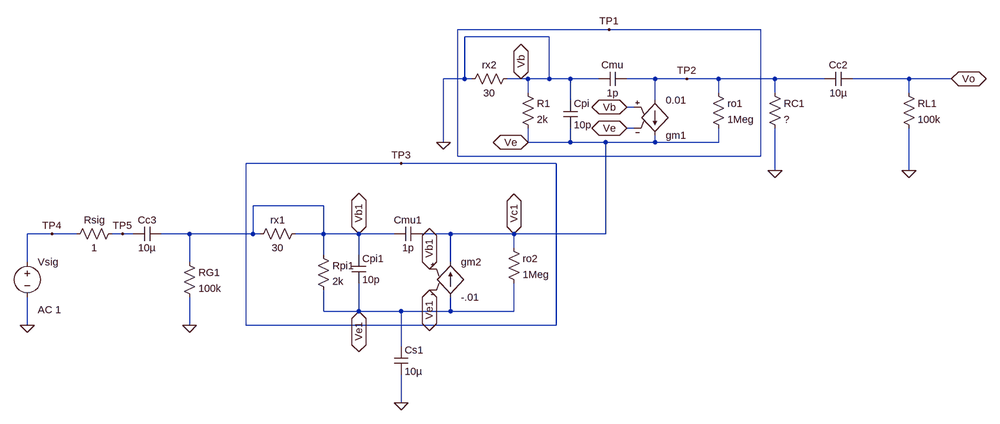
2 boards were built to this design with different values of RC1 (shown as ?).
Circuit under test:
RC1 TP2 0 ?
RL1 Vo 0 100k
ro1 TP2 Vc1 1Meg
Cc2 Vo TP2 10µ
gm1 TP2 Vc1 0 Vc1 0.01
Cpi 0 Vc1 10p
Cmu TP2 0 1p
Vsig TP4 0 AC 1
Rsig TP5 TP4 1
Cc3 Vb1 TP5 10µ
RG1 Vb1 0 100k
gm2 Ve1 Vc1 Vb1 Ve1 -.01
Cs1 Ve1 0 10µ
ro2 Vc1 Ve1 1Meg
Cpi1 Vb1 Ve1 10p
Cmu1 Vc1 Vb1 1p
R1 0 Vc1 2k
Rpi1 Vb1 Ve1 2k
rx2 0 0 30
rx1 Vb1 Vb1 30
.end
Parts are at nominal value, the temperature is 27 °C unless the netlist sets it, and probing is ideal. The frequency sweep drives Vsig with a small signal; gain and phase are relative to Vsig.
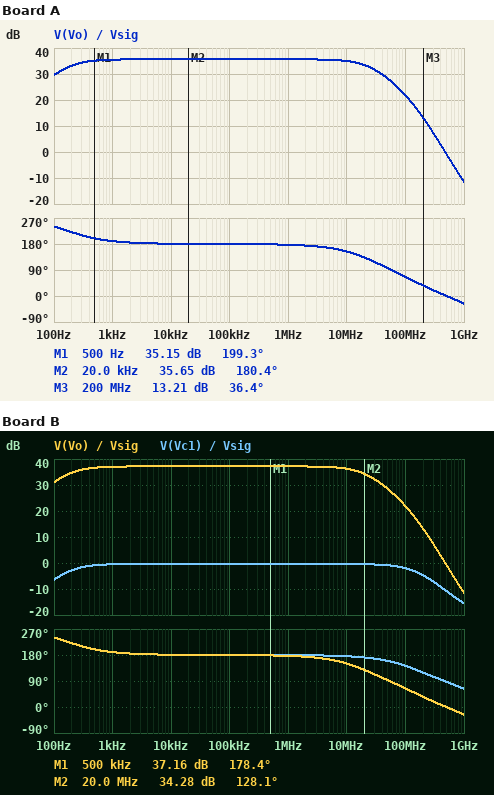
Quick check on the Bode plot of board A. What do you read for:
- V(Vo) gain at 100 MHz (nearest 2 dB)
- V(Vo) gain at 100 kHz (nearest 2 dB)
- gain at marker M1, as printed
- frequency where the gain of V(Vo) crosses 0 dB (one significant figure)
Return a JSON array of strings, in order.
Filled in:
["22 dB", "36 dB", "35.15 dB", "500 MHz"]
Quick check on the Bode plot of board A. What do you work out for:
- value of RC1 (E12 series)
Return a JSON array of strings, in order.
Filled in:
["6.8 kΩ"]
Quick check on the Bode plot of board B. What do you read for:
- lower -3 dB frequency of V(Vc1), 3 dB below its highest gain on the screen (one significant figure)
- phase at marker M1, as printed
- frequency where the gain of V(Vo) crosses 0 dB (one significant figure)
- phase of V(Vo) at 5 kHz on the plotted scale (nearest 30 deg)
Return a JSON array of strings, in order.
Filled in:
["200 Hz", "178.4 deg", "500 MHz", "180 deg"]
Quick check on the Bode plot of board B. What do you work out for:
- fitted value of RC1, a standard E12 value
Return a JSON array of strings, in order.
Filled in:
["8.2 kΩ"]
